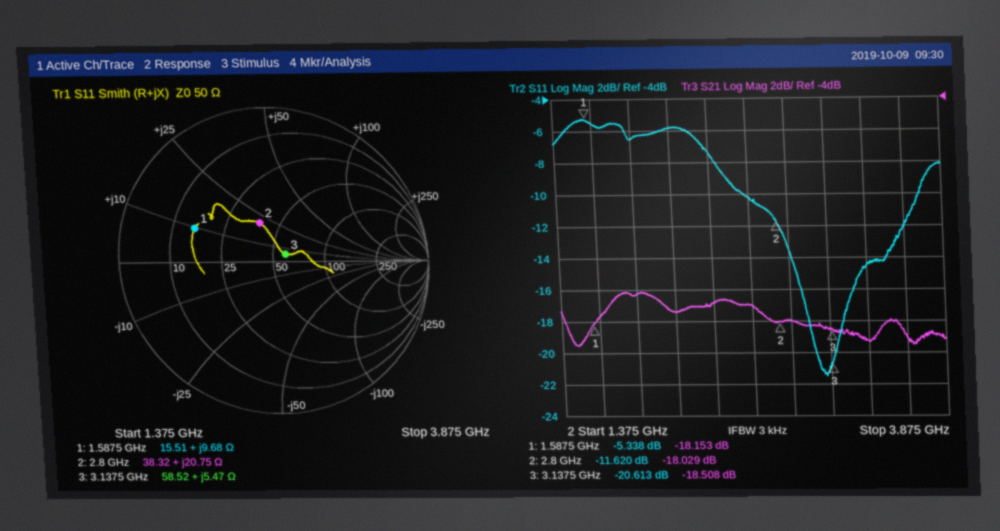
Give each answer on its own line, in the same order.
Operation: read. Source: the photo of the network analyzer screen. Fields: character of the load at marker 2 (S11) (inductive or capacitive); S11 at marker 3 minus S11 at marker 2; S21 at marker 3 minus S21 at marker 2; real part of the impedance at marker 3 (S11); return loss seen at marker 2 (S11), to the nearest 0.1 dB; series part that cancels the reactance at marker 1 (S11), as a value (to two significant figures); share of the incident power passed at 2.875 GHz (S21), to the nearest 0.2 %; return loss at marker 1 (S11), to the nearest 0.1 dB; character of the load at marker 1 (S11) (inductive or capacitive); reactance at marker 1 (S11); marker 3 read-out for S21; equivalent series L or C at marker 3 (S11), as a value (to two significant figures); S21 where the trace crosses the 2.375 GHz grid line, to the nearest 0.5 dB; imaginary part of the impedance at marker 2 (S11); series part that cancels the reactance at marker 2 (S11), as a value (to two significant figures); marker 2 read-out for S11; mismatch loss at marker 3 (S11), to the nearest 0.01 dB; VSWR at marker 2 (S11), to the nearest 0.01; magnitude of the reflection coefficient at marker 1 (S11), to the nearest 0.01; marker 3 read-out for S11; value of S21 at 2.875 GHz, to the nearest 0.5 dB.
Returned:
inductive
-8.993 dB
-0.479 dB
58.52 Ω
11.6 dB
10 pF
1.6 %
5.3 dB
inductive
+9.68 Ω
-18.508 dB
280 pH
-17.0 dB
+20.75 Ω
2.7 pF
-11.620 dB
0.04 dB
1.71
0.54
-20.613 dB
-18.0 dB
